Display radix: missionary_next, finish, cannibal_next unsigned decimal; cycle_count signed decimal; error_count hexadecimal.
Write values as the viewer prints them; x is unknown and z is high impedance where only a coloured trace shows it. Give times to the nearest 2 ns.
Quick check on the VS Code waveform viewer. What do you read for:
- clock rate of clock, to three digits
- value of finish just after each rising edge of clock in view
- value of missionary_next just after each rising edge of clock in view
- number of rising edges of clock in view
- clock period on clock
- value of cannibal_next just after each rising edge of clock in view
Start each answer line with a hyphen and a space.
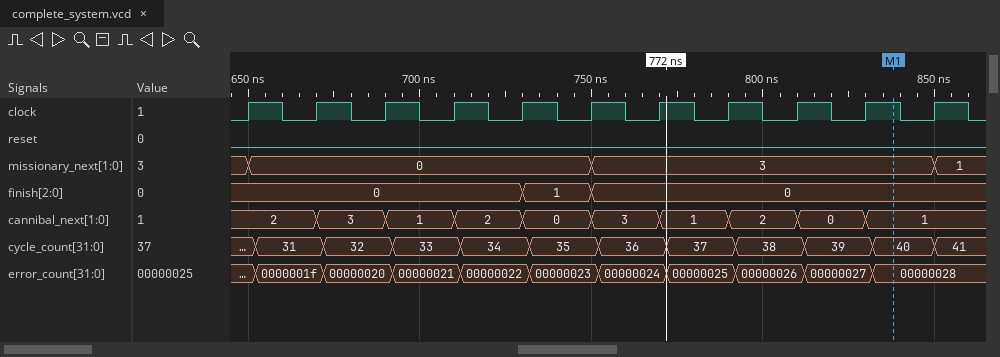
- 50.0 MHz
- 0, 0, 0, 0, 1, 0, 0, 0, 0, 0, 0
- 0, 0, 0, 0, 0, 3, 3, 3, 3, 3, 1
- 11
- 20 ns
- 2, 3, 1, 2, 0, 3, 1, 2, 0, 1, 1
